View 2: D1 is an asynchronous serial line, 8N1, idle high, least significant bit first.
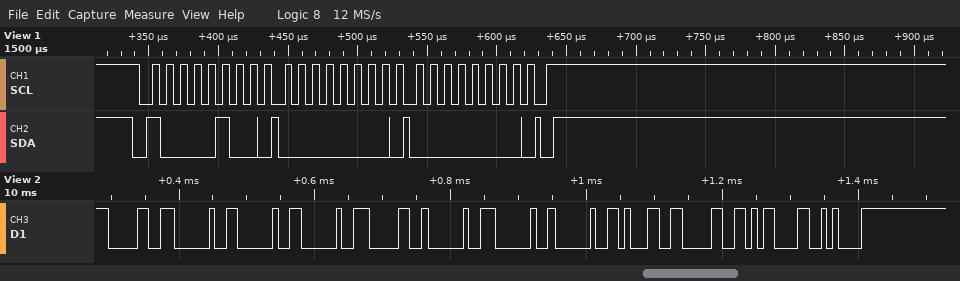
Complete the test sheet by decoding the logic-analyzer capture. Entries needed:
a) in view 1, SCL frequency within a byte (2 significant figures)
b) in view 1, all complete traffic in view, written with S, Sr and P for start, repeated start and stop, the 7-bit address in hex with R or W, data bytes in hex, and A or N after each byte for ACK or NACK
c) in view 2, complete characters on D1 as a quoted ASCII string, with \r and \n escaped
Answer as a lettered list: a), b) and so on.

a) 100 kHz
b) S 42W A 00 A 00 A P
c) "0   0   10\r\n"
